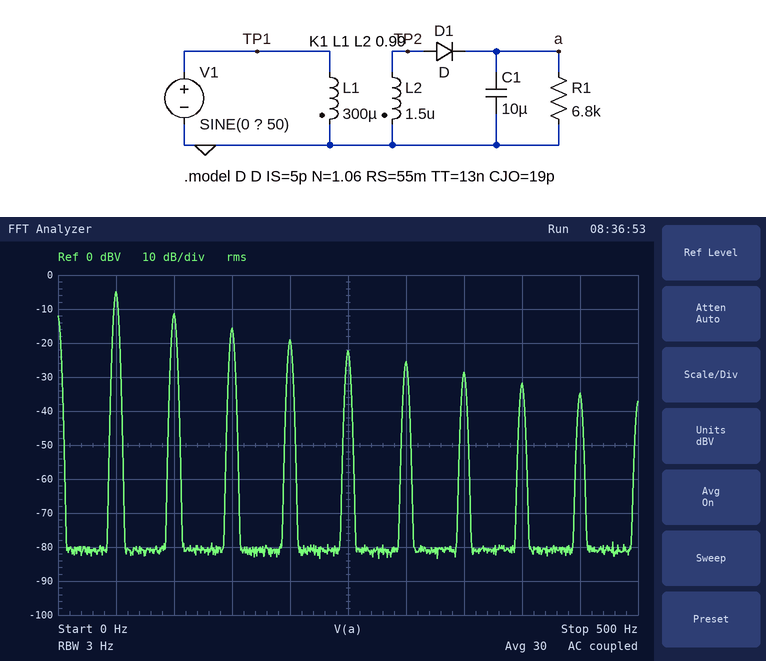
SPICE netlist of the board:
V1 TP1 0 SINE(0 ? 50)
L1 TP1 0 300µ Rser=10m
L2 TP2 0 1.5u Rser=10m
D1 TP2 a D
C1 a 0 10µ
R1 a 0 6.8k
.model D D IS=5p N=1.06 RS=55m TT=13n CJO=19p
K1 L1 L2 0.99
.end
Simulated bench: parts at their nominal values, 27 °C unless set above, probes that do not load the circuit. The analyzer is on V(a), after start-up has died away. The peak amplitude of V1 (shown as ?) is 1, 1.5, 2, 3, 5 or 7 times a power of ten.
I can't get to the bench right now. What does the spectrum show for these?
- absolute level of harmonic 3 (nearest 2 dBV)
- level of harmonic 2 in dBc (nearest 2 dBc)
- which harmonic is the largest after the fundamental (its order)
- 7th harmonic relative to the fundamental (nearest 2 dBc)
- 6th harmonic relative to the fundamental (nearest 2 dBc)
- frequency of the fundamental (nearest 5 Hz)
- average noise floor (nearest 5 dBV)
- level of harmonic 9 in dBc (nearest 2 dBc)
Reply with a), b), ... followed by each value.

a) -16 dBV
b) -6 dBc
c) 2
d) -24 dBc
e) -20 dBc
f) 50 Hz
g) -80 dBV
h) -30 dBc
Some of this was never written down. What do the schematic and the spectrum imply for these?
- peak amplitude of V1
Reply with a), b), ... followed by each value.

a) 150 V
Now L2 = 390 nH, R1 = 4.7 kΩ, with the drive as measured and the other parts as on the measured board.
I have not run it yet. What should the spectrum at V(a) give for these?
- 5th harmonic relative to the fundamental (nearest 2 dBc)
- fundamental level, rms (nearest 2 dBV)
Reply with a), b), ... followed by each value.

a) -18 dBc
b) -8 dBV
